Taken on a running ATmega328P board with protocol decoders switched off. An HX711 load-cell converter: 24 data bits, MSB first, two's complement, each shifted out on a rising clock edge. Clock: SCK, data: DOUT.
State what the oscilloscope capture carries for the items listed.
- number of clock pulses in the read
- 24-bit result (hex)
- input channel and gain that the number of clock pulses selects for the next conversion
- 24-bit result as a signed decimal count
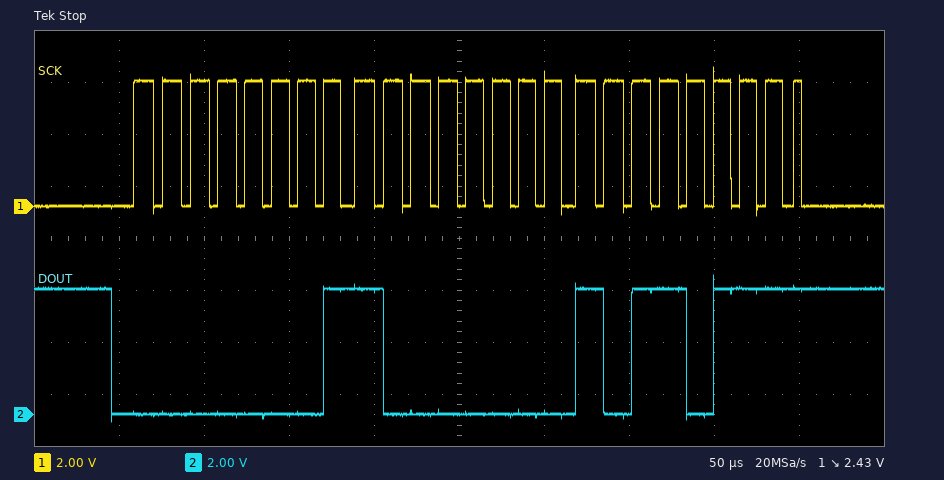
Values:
25
0x0180B7
channel A, gain 128
98487
